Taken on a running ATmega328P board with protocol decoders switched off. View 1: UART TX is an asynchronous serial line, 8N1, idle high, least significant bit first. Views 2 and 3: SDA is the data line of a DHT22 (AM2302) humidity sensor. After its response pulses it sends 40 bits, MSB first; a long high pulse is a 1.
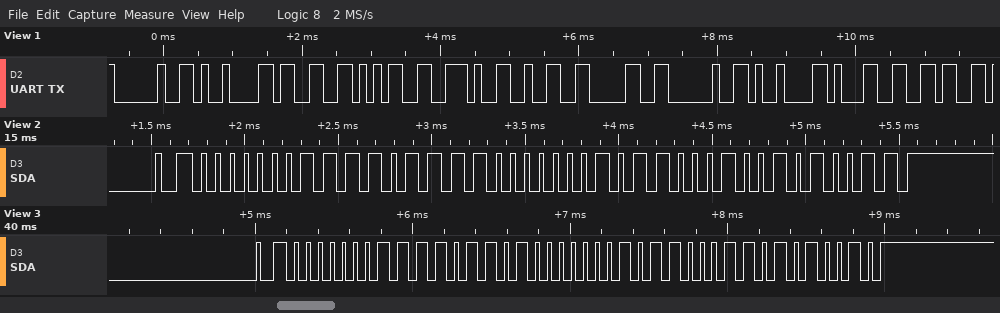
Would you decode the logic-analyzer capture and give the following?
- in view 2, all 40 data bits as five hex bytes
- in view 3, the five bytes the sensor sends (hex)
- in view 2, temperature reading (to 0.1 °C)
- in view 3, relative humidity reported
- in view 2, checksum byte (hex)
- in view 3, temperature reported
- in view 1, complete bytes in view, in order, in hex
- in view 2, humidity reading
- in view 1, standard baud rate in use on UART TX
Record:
01 EF 01 62 53
01 ED 01 63 52
35.4 °C
49.3 %
0x53
35.5 °C
0x20 0x09 0x33 0x35 0x2E 0x32 0x30 0x20 0x09 0x31 0x36
49.5 %
9600 baud
